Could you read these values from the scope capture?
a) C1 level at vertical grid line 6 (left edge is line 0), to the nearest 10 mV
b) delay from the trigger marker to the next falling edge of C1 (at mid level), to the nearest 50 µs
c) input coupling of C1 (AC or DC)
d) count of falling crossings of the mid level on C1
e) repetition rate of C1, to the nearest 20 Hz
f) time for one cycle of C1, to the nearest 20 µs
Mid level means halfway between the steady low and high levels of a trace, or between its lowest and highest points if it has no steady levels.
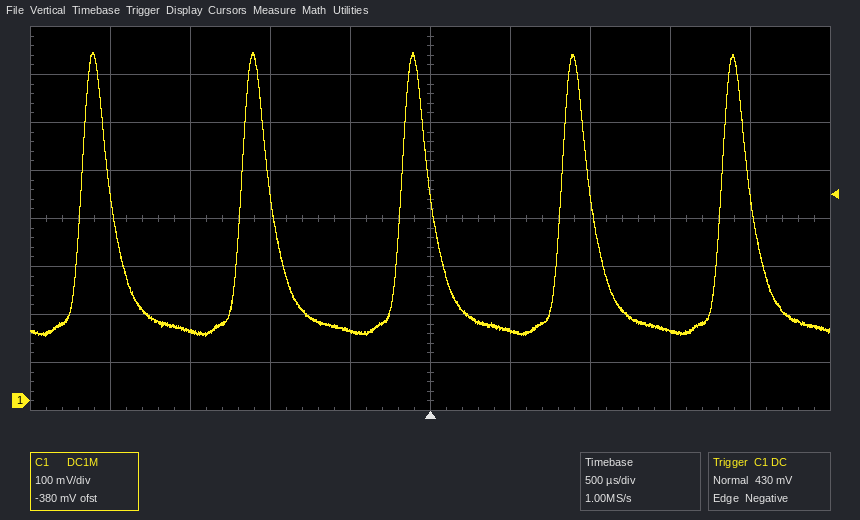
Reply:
150 mV
1.00 ms
DC
5
1.00 kHz
1.00 ms
